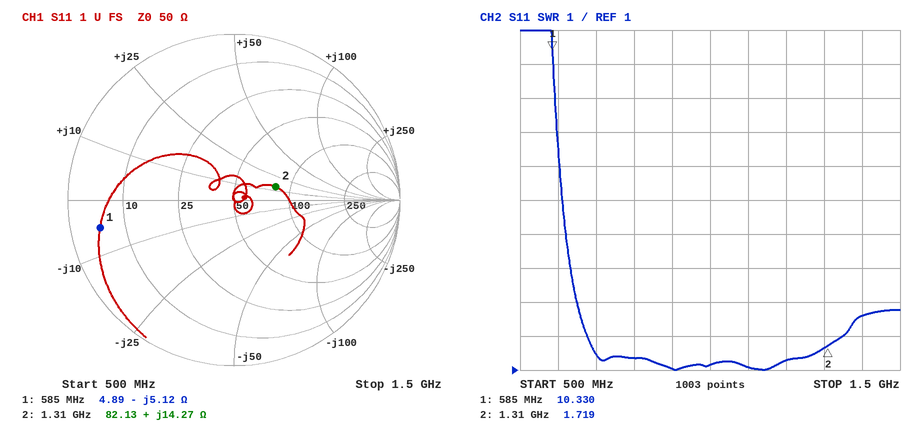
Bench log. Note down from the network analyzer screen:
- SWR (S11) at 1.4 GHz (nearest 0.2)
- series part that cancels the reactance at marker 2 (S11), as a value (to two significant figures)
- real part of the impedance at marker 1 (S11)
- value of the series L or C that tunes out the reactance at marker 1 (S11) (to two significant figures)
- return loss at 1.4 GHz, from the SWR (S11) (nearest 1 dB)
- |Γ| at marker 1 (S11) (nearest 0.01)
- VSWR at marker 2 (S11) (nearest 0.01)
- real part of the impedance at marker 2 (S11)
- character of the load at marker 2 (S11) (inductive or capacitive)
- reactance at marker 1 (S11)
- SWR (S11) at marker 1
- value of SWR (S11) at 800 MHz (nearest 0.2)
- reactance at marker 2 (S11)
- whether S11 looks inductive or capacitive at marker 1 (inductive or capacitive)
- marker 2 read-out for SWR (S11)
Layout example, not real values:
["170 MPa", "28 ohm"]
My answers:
["2.6", "8.5 pF", "4.89 Ω", "1.4 nH", "7 dB", "0.82", "1.72", "82.13 Ω", "inductive", "-5.12 Ω", "10.330", "1.4", "+14.27 Ω", "capacitive", "1.719"]
